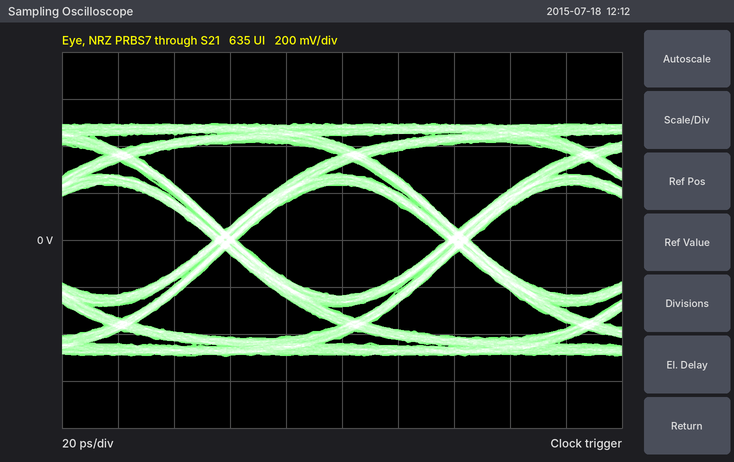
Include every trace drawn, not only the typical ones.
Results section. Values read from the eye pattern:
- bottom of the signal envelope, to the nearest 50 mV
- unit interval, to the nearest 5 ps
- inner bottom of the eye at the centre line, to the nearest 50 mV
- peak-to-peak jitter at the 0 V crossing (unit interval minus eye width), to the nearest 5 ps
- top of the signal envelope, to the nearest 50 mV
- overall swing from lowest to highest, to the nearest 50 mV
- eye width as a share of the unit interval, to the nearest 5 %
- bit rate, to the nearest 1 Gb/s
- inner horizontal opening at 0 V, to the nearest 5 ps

-500 mV
85 ps
-250 mV
10 ps
500 mV
1.00 V
90 %
12 Gb/s
75 ps
